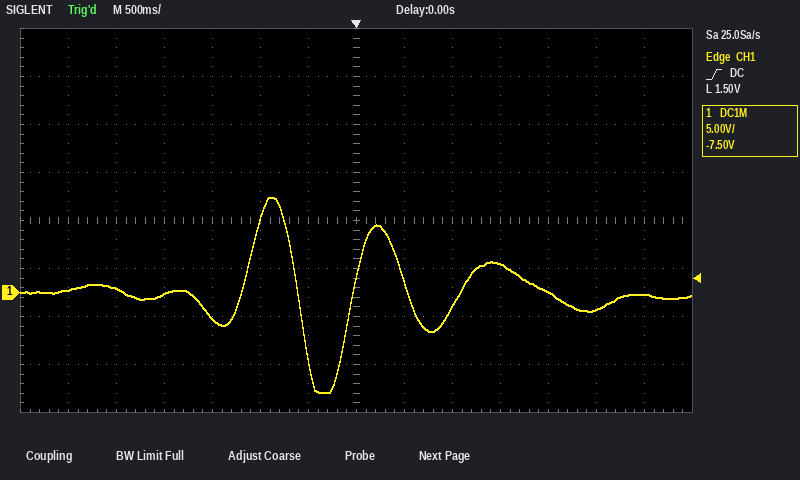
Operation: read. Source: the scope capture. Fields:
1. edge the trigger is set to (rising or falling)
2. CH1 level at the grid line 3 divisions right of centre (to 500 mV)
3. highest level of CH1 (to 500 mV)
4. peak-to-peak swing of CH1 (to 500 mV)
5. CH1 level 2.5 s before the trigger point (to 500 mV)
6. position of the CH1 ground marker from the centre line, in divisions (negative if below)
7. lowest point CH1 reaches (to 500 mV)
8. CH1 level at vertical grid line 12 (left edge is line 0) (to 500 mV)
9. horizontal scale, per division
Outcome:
rising
3.0 V
10.0 V
20.5 V
500 mV
-1.5 div
-10.5 V
-2.0 V
500 ms
